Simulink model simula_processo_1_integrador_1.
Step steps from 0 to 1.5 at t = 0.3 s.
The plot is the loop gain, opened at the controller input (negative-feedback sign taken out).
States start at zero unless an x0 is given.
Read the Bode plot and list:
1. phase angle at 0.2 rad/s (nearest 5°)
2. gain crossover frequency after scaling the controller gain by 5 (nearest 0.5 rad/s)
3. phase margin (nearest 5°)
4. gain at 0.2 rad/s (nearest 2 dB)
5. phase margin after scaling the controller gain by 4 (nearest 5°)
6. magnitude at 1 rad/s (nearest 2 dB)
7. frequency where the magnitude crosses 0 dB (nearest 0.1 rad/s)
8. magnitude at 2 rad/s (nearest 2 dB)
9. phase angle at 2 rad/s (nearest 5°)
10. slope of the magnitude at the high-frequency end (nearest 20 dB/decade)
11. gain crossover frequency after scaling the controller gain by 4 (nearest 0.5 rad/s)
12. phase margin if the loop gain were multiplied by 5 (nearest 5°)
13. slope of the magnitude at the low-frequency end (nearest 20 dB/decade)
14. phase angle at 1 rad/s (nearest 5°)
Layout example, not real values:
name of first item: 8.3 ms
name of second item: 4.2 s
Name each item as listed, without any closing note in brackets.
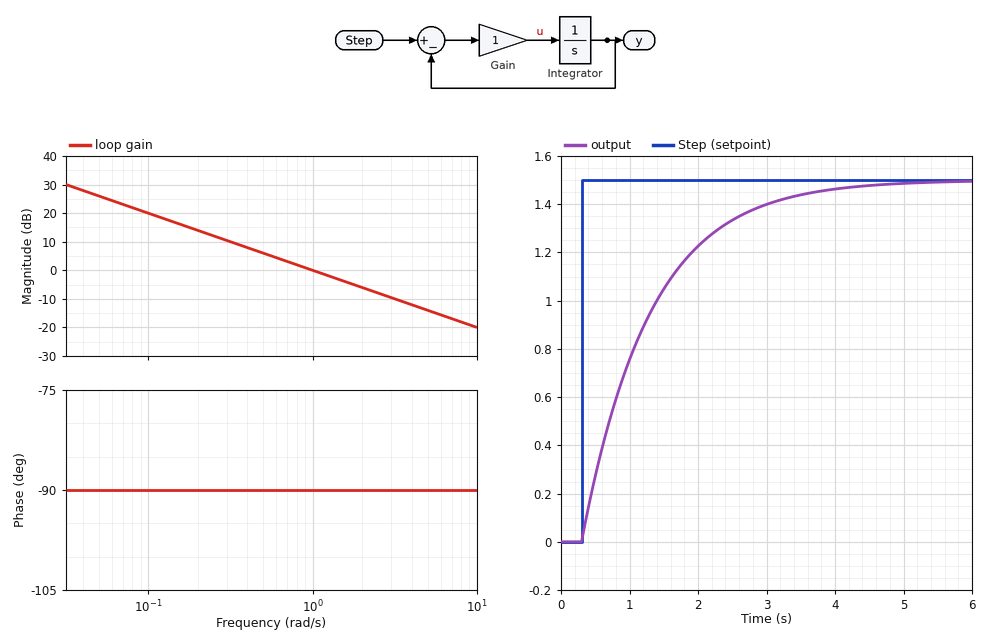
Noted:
phase angle at 0.2 rad/s: -90°
gain crossover frequency after scaling the controller gain by 5: 5.0 rad/s
phase margin: 90°
gain at 0.2 rad/s: 14 dB
phase margin after scaling the controller gain by 4: 90°
magnitude at 1 rad/s: 0 dB
frequency where the magnitude crosses 0 dB: 1.0 rad/s
magnitude at 2 rad/s: -6 dB
phase angle at 2 rad/s: -90°
slope of the magnitude at the high-frequency end: -20 dB/decade
gain crossover frequency after scaling the controller gain by 4: 4.0 rad/s
phase margin if the loop gain were multiplied by 5: 90°
slope of the magnitude at the low-frequency end: -20 dB/decade
phase angle at 1 rad/s: -90°
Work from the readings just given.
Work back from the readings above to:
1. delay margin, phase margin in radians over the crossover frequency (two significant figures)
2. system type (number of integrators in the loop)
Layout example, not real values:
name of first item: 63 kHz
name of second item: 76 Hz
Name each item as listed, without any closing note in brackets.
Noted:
delay margin, phase margin in radians over the crossover frequency: 1.6 s
system type: 1
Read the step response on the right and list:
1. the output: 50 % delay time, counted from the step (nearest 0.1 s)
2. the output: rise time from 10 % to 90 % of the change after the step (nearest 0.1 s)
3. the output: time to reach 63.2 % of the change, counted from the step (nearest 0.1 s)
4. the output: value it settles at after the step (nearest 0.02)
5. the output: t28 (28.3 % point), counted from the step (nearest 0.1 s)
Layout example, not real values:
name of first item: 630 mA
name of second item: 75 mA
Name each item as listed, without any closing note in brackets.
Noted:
the output: 50 % delay time, counted from the step: 0.7 s
the output: rise time from 10 % to 90 % of the change after the step: 2.2 s
the output: time to reach 63.2 % of the change, counted from the step: 1.0 s
the output: value it settles at after the step: 1.50
the output: t28 (28.3 % point), counted from the step: 0.3 s
